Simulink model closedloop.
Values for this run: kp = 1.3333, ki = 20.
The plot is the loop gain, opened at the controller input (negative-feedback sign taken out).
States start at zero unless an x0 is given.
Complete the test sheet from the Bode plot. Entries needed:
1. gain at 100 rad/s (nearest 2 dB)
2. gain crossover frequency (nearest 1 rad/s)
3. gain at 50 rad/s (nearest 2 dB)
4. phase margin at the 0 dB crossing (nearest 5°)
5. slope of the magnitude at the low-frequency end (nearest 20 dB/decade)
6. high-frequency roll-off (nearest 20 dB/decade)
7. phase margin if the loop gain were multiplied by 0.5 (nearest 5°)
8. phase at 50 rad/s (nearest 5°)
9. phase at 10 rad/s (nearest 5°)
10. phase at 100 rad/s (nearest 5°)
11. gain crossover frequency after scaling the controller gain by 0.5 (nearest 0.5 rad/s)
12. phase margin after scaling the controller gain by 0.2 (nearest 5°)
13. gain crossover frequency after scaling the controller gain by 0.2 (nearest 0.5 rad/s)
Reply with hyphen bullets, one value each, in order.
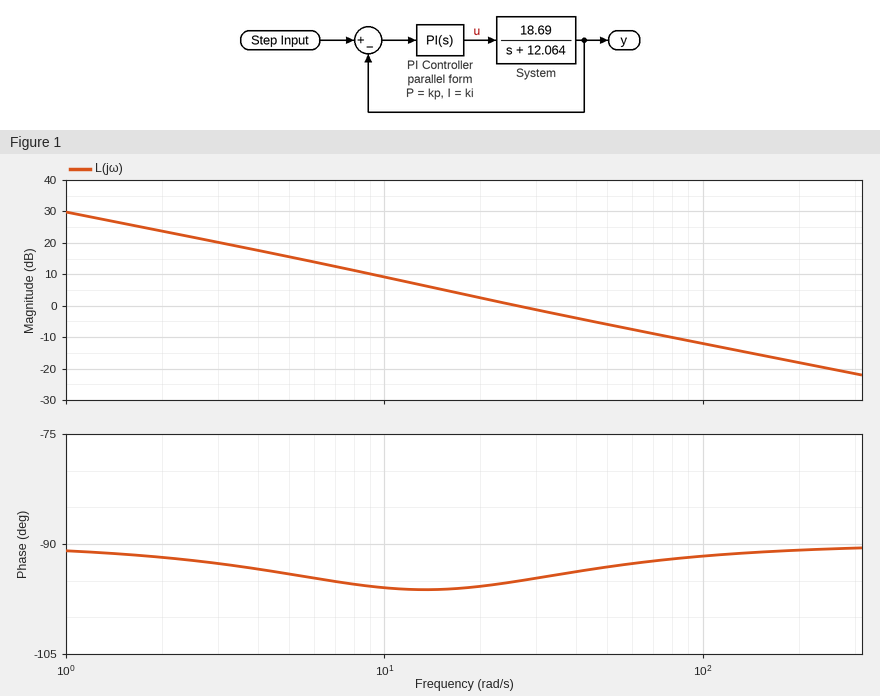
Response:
- -12 dB
- 26 rad/s
- -6 dB
- 85°
- -20 dB/decade
- -20 dB/decade
- 85°
- -95°
- -95°
- -90°
- 14.0 rad/s
- 85°
- 6.0 rad/s
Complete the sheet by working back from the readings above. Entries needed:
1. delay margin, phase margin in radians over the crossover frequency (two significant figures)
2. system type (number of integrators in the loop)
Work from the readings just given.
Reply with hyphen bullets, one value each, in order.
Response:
- 0.057 s
- 1
